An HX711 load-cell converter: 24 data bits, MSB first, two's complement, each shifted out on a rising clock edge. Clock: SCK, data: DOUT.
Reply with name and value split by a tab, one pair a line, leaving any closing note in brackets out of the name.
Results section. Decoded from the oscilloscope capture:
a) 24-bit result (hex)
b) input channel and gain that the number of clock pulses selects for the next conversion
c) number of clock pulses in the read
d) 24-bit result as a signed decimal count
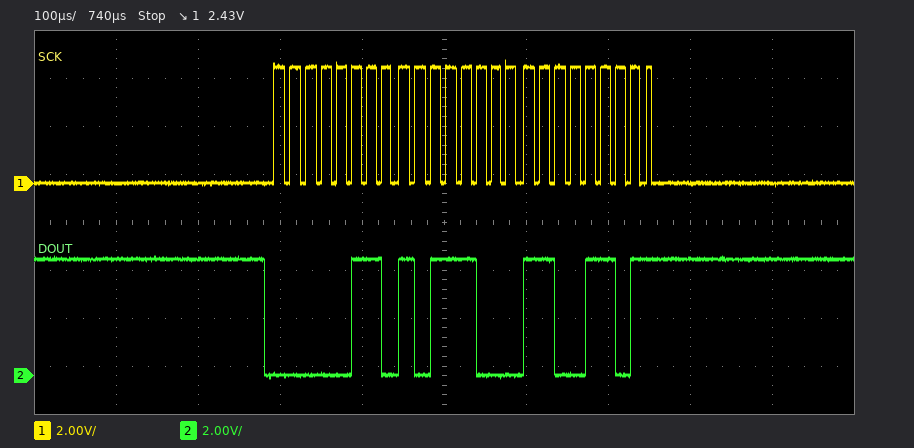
24-bit result	0x06B8CD
input channel and gain that the number of clock pulses selects for the next conversion	channel A, gain 128
number of clock pulses in the read	25
24-bit result as a signed decimal count	440525
